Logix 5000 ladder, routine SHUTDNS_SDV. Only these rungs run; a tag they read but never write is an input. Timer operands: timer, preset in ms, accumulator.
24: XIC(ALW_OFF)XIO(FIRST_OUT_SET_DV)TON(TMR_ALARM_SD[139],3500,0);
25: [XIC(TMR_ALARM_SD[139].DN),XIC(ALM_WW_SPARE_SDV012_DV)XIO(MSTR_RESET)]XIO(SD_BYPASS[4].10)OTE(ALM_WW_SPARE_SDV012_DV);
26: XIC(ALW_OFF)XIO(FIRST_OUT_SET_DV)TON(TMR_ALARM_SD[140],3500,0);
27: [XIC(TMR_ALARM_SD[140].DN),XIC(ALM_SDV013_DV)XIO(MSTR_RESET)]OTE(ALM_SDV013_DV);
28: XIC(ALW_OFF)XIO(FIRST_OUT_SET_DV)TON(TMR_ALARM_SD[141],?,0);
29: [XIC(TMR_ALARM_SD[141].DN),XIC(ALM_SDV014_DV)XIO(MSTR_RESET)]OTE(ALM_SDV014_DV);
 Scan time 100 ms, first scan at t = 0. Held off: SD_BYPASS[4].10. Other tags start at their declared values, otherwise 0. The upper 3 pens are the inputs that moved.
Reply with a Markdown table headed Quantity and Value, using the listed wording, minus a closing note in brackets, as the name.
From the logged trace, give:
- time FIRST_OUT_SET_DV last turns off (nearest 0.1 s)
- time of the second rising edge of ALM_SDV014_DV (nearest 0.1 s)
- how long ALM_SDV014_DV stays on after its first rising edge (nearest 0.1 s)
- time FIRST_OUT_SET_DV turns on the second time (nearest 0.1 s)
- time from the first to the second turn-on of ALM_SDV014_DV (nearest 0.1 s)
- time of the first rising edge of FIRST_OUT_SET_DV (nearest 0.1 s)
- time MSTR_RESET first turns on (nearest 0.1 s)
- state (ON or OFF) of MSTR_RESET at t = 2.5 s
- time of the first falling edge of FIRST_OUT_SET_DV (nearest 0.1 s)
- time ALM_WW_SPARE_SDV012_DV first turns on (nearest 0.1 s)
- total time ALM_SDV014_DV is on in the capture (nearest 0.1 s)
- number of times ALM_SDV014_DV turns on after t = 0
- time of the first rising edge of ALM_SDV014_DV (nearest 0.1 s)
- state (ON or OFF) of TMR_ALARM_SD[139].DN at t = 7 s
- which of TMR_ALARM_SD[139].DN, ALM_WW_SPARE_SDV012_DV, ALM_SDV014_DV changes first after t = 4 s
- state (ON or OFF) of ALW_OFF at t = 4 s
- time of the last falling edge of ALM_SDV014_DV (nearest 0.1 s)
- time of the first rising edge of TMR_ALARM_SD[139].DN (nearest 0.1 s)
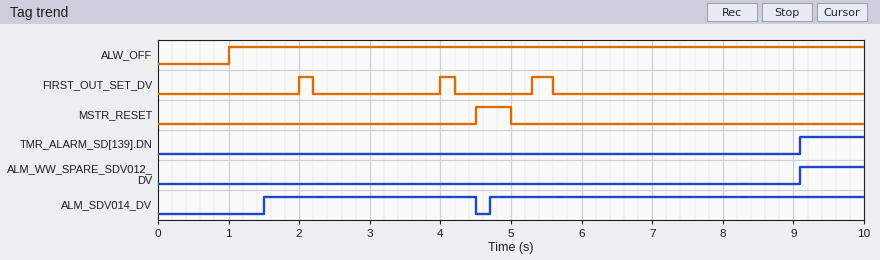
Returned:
| Quantity | Value |
|---|---|
| time FIRST_OUT_SET_DV last turns off | 5.6 s |
| time of the second rising edge of ALM_SDV014_DV | 4.7 s |
| how long ALM_SDV014_DV stays on after its first rising edge | 3.0 s |
| time FIRST_OUT_SET_DV turns on the second time | 4.0 s |
| time from the first to the second turn-on of ALM_SDV014_DV | 3.2 s |
| time of the first rising edge of FIRST_OUT_SET_DV | 2.0 s |
| time MSTR_RESET first turns on | 4.5 s |
| state (ON or OFF) of MSTR_RESET at t = 2.5 s | OFF |
| time of the first falling edge of FIRST_OUT_SET_DV | 2.2 s |
| time ALM_WW_SPARE_SDV012_DV first turns on | 9.1 s |
| total time ALM_SDV014_DV is on in the capture | 8.3 s |
| number of times ALM_SDV014_DV turns on after t = 0 | 2 |
| time of the first rising edge of ALM_SDV014_DV | 1.5 s |
| state (ON or OFF) of TMR_ALARM_SD[139].DN at t = 7 s | OFF |
| which of TMR_ALARM_SD[139].DN, ALM_WW_SPARE_SDV012_DV, ALM_SDV014_DV changes first after t = 4 s | ALM_SDV014_DV |
| state (ON or OFF) of ALW_OFF at t = 4 s | ON |
| time of the last falling edge of ALM_SDV014_DV | 4.5 s |
| time of the first rising edge of TMR_ALARM_SD[139].DN | 9.1 s |
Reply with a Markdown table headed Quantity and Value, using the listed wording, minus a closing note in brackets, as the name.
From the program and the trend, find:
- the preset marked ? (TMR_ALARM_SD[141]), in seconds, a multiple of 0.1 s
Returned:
| Quantity | Value |
|---|---|
| the preset marked ? (TMR_ALARM_SD[141]), in seconds, a multiple of 0.1 s | 0.5 s |
